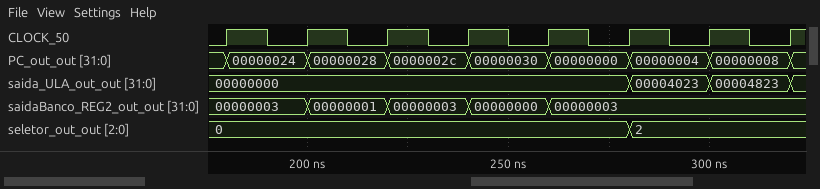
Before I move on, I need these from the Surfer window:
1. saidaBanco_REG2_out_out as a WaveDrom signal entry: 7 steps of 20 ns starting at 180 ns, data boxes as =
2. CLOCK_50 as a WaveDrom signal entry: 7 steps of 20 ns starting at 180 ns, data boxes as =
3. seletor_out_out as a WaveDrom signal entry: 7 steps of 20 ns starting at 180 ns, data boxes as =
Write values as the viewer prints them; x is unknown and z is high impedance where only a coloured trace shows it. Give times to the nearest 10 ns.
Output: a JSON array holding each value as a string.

["{name: 'saidaBanco_REG2_out_out', wave: '=====..', data: '00000003 00000001 00000003 00000000 00000003'}", "{name: 'CLOCK_50', wave: 'p......'}", "{name: 'seletor_out_out', wave: '=....=.', data: '0 2'}"]
